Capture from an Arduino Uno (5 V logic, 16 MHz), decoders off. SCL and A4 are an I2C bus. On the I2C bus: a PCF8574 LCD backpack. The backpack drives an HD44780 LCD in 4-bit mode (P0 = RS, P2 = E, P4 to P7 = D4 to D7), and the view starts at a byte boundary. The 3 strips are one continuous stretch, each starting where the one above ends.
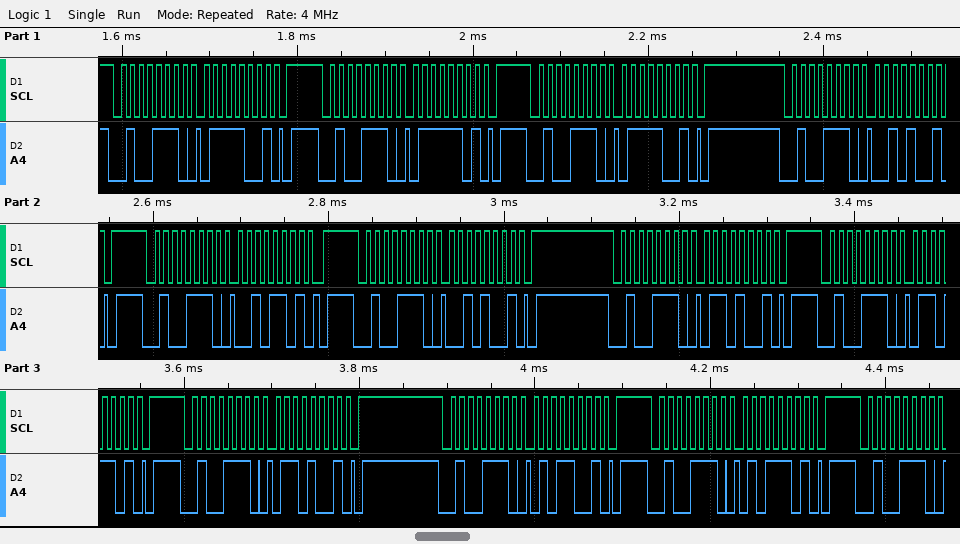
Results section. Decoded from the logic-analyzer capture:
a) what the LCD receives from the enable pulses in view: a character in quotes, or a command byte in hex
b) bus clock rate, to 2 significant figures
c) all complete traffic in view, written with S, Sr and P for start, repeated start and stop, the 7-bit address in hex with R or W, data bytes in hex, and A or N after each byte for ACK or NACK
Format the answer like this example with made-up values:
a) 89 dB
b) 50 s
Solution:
a) 'r'
b) 100 kHz
c) S 27W A 79 A P S 27W A 7D A P S 27W A 79 A P S 27W A 29 A P S 27W A 2D A P S 27W A 29 A P S 27W A 69 A P S 27W A 6D A P S 27W A 69 A P S 27W A 59 A P S 27W A 5D A P S 27W A
